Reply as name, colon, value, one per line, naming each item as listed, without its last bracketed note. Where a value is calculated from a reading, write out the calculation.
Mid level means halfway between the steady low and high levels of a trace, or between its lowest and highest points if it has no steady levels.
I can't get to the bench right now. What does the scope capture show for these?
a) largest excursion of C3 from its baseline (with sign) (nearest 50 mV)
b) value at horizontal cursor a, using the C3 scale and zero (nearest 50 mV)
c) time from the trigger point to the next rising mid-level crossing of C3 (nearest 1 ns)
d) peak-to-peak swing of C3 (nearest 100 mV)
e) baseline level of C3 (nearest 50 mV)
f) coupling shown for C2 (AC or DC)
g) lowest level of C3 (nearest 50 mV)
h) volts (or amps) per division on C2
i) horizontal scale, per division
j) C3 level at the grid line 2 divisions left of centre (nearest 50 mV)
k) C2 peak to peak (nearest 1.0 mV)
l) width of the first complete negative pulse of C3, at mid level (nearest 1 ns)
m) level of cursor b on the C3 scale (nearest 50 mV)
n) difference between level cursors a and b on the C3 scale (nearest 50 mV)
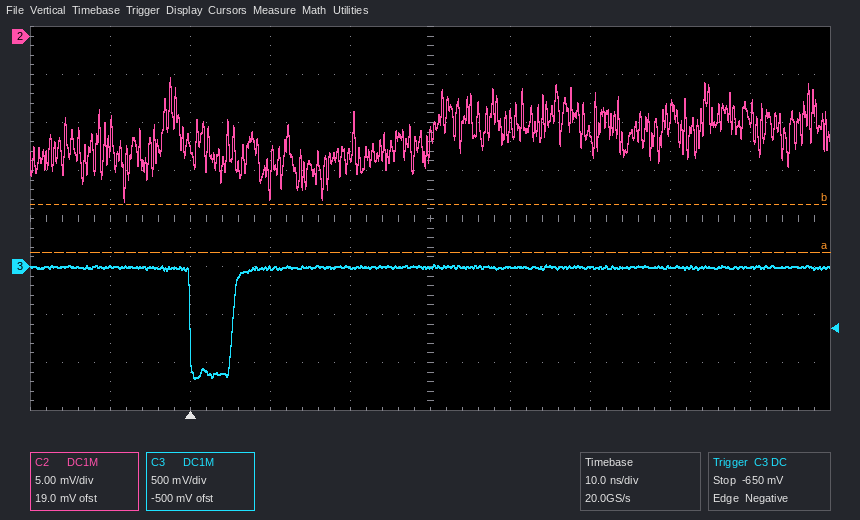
largest excursion of C3 from its baseline (with sign): -1.15 V − (0 mV) = -1.15 V
value at horizontal cursor a, using the C3 scale and zero: 150 mV
time from the trigger point to the next rising mid-level crossing of C3: 5 ns
peak-to-peak swing of C3: 1.20 V
baseline level of C3: 0 mV
coupling shown for C2: DC
lowest level of C3: -1.15 V
volts (or amps) per division on C2: 5 mV
horizontal scale, per division: 10 ns
C3 level at the grid line 2 divisions left of centre: 0 mV
C2 peak to peak: 13.0 mV
width of the first complete negative pulse of C3, at mid level: 5 ns
level of cursor b on the C3 scale: 650 mV
difference between level cursors a and b on the C3 scale: 500 mV
